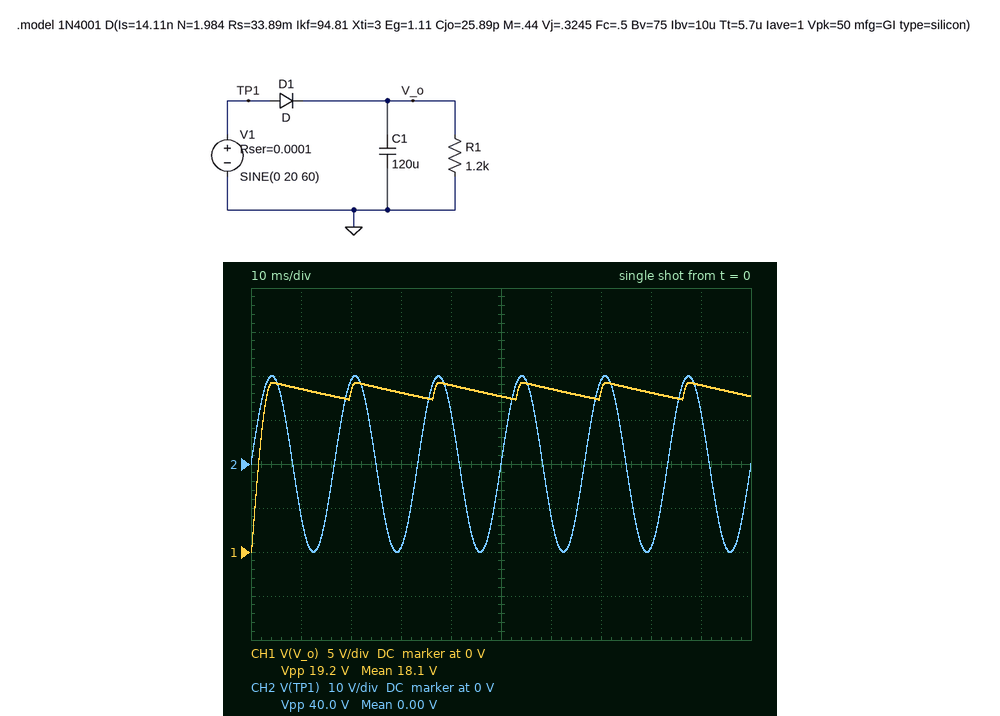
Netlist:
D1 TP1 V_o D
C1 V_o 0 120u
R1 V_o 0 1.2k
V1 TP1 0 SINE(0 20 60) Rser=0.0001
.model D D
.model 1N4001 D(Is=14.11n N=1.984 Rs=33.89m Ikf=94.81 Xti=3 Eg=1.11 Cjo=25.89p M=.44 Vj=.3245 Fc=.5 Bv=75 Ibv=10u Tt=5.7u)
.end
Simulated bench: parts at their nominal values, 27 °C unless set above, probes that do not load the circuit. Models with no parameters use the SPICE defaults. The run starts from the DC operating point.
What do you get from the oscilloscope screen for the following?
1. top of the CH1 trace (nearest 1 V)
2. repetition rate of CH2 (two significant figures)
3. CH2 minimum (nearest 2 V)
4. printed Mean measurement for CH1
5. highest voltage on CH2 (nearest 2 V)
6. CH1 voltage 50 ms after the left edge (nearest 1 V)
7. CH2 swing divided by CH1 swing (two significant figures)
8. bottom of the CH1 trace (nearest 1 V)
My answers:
19 V
60 Hz
-20 V
18.1 V
20 V
18 V
2.1
0 V
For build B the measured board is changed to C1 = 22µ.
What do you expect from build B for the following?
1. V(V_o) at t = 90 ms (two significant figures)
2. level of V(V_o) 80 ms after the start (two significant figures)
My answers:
18 V
14 V
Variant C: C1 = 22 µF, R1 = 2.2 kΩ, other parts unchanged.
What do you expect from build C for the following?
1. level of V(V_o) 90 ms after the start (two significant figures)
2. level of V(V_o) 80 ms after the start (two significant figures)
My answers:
18 V
16 V
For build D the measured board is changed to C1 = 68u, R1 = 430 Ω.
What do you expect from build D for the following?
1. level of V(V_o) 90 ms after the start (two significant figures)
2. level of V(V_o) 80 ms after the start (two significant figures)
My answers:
18 V
14 V
